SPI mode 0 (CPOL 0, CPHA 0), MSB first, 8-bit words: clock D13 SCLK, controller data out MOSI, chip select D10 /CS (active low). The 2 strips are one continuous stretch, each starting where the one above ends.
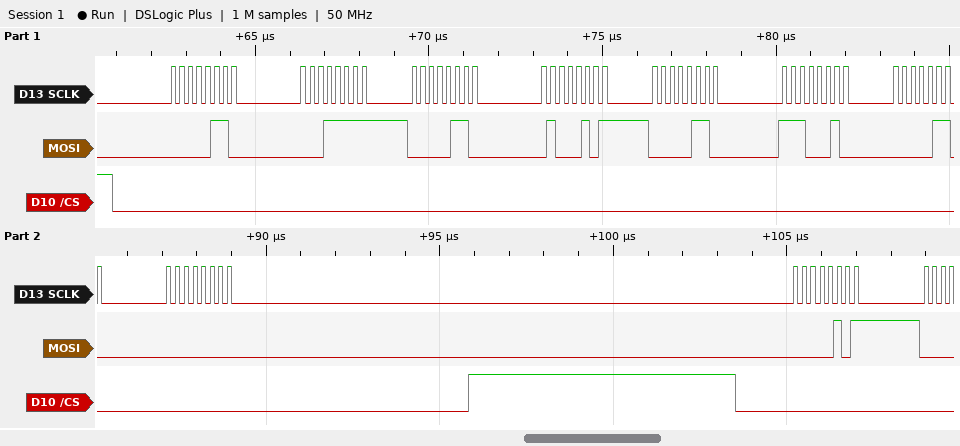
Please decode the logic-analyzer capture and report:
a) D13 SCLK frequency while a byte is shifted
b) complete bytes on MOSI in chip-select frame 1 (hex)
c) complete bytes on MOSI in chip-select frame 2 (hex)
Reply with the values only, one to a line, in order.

4 MHz
0x06 0x1F 0x06 0x45 0x06 0xE2 0x06 0x00
0x05
